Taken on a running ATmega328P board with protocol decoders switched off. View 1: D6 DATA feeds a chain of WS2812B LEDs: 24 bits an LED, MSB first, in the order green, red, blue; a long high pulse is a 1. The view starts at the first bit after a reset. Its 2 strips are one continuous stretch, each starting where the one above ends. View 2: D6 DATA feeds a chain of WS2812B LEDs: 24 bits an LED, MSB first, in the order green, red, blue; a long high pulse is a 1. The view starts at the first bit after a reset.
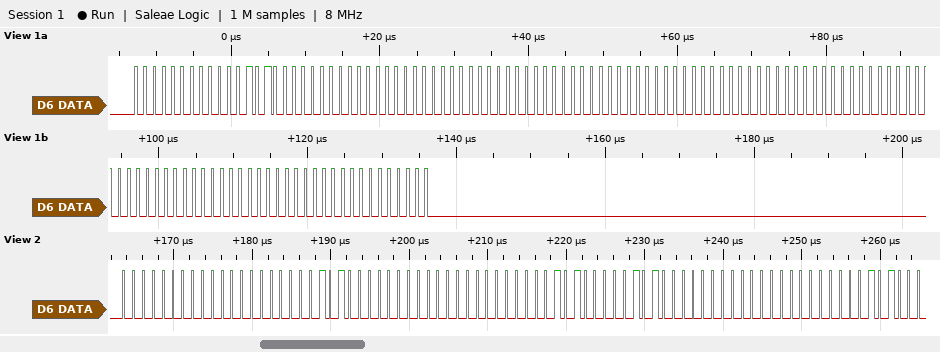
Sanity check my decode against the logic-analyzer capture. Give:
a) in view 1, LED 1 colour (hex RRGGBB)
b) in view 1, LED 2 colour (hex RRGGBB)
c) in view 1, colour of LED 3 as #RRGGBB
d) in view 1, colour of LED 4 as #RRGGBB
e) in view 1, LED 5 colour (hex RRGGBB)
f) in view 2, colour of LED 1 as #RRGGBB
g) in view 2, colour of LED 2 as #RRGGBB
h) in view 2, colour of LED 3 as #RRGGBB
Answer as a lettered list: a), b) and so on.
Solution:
a) #0A0000
b) #000000
c) #000000
d) #000000
e) #000000
f) #00000A
g) #00000A
h) #000A00
